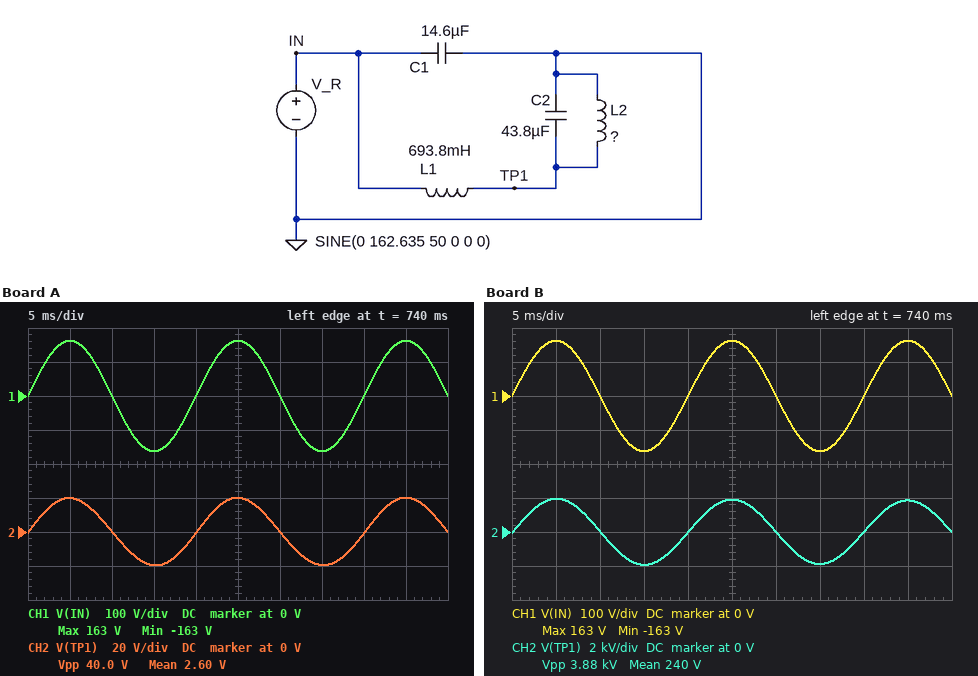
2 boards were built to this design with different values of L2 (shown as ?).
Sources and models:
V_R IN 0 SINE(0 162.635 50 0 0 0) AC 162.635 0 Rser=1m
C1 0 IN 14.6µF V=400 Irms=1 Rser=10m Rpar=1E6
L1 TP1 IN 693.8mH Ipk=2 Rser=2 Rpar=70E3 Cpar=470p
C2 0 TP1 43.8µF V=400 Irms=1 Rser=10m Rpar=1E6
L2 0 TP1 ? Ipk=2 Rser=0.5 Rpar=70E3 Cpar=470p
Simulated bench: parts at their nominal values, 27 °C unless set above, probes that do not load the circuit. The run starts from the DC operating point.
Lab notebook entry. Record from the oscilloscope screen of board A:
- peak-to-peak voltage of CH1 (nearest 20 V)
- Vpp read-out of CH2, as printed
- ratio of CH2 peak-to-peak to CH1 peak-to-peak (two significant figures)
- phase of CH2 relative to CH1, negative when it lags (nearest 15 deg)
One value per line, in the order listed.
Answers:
320 V
40.0 V
0.12
0 deg
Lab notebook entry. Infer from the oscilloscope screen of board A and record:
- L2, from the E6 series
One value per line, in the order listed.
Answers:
68 mH
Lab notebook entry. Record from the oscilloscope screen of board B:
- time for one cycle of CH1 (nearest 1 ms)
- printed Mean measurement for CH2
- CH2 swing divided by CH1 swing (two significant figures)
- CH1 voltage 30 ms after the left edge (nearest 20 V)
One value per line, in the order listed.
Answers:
20 ms
240 V
12
0 V
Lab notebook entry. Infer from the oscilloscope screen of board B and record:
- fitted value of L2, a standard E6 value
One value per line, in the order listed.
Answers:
330 mH
